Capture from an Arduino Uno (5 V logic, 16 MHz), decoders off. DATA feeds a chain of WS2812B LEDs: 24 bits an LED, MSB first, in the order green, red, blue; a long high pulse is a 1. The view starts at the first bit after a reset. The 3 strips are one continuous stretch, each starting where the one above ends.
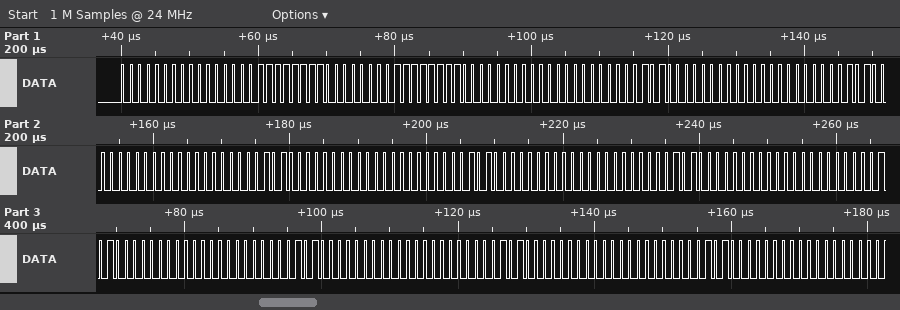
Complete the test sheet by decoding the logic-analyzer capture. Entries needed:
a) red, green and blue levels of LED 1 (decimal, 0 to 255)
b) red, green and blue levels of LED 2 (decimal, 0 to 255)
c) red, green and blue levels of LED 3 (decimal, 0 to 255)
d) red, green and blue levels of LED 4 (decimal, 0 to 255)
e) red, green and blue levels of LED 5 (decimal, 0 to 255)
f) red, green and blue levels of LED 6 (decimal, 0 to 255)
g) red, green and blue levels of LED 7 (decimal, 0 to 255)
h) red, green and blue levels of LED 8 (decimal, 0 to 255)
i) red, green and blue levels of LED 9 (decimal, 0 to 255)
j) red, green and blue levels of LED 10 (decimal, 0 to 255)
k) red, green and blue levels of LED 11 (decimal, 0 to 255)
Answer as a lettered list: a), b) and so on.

a) 0, 0, 255
b) 255, 0, 0
c) 5, 0, 0
d) 5, 0, 0
e) 5, 0, 0
f) 5, 0, 0
g) 5, 0, 0
h) 5, 0, 0
i) 5, 0, 0
j) 5, 0, 0
k) 5, 0, 0
